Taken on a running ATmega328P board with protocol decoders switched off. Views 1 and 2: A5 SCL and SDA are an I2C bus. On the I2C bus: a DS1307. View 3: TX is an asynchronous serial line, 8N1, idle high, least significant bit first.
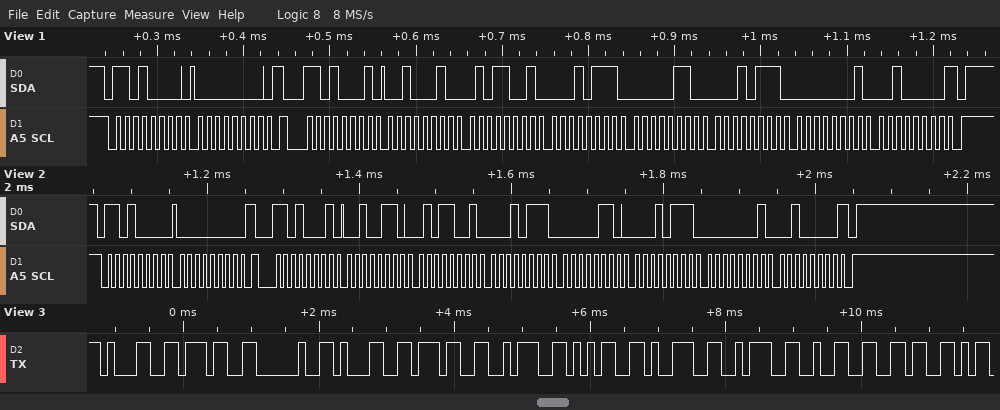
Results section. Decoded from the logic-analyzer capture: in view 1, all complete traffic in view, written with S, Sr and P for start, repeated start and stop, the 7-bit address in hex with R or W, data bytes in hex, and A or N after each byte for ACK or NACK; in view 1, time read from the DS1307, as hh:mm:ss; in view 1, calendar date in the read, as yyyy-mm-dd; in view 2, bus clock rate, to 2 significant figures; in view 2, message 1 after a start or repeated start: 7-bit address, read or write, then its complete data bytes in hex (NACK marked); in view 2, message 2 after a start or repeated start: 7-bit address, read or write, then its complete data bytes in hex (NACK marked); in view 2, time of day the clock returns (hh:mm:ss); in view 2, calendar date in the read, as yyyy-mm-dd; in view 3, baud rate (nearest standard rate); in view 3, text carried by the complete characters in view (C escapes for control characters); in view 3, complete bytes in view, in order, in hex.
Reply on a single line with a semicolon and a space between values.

S 68W A 00 A Sr 68R A 22 A 59 A 17 A 06 A 17 A 01 A 20 N P; 17:59:22; 2020-01-17; 100 kHz; 0x68 write: 00; 0x68 read: 26 59 17 06 17 01 20 NACK; 17:59:26; 2020-01-17; 9600 baud; "17 17:59:26"; 0x31 0x37 0x20 0x31 0x37 0x3A 0x35 0x39 0x3A 0x32 0x36
